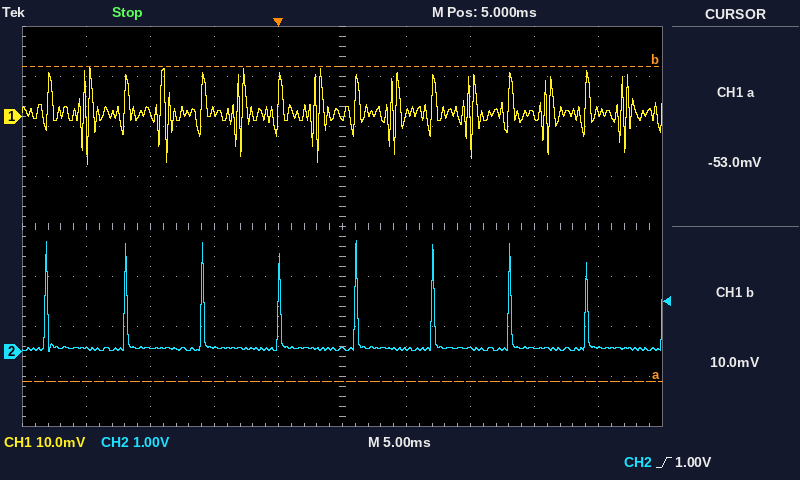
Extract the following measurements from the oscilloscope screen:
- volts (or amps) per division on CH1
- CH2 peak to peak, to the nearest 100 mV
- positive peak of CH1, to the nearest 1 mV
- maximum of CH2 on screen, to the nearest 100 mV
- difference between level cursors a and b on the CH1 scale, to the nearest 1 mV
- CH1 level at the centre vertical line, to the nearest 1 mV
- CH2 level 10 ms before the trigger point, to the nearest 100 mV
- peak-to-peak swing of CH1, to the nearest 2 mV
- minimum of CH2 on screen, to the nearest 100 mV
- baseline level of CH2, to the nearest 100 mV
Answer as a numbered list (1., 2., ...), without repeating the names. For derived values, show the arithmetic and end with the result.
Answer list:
1. 10 mV
2. 2.2 V − (0.0 V) = 2.2 V
3. 10 mV
4. 2.2 V
5. 63 mV
6. 0 mV
7. 100 mV
8. 20 mV
9. 0.0 V
10. 100 mV
